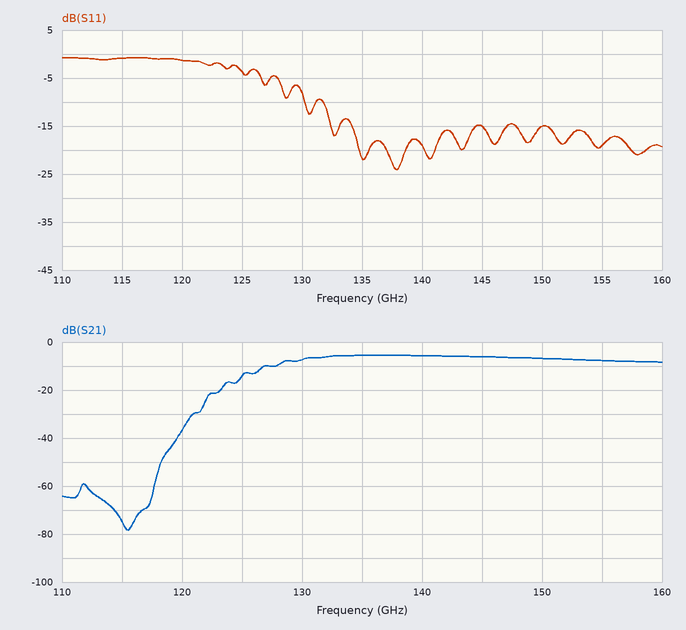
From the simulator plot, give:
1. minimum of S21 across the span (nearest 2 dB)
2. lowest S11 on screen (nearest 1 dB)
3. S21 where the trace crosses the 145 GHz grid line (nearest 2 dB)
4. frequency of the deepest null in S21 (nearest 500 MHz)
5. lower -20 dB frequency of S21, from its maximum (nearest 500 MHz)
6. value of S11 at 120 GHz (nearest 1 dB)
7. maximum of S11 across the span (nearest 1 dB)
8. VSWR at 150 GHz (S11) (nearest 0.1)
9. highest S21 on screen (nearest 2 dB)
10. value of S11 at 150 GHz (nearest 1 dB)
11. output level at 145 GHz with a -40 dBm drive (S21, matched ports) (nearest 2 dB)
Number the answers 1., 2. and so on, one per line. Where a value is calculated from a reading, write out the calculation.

1. -78 dB
2. -24 dB
3. -6 dB
4. 115.5 GHz
5. 122.0 GHz
6. -1 dB
7. -1 dB
8. |Γ| = 10^(-15/20) = 0.1778; VSWR = (1 + 0.1778)/(1 − 0.1778) ≈ 1.4
9. -6 dB
10. -15 dB
11. -40 dBm + (-6 dB) = -46 dBm
